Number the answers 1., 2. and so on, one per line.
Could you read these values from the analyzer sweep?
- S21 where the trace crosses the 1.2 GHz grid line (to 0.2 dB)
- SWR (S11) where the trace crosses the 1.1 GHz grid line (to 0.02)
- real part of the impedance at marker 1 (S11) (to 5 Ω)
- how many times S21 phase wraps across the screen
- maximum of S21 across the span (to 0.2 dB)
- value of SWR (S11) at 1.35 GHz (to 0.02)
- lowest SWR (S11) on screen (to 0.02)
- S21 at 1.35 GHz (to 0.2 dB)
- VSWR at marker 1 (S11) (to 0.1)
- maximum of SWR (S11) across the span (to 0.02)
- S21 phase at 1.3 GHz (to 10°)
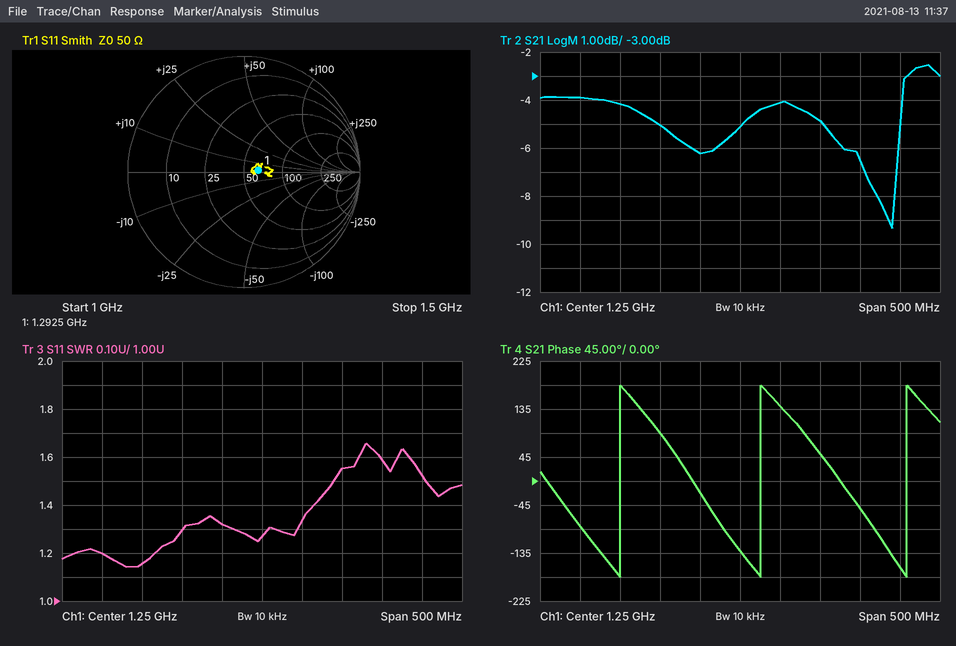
1. -6.2 dB
2. 1.16
3. 65 Ω
4. 3
5. -2.6 dB
6. 1.56
7. 1.14
8. -4.8 dB
9. 1.3
10. 1.66
11. 140°
